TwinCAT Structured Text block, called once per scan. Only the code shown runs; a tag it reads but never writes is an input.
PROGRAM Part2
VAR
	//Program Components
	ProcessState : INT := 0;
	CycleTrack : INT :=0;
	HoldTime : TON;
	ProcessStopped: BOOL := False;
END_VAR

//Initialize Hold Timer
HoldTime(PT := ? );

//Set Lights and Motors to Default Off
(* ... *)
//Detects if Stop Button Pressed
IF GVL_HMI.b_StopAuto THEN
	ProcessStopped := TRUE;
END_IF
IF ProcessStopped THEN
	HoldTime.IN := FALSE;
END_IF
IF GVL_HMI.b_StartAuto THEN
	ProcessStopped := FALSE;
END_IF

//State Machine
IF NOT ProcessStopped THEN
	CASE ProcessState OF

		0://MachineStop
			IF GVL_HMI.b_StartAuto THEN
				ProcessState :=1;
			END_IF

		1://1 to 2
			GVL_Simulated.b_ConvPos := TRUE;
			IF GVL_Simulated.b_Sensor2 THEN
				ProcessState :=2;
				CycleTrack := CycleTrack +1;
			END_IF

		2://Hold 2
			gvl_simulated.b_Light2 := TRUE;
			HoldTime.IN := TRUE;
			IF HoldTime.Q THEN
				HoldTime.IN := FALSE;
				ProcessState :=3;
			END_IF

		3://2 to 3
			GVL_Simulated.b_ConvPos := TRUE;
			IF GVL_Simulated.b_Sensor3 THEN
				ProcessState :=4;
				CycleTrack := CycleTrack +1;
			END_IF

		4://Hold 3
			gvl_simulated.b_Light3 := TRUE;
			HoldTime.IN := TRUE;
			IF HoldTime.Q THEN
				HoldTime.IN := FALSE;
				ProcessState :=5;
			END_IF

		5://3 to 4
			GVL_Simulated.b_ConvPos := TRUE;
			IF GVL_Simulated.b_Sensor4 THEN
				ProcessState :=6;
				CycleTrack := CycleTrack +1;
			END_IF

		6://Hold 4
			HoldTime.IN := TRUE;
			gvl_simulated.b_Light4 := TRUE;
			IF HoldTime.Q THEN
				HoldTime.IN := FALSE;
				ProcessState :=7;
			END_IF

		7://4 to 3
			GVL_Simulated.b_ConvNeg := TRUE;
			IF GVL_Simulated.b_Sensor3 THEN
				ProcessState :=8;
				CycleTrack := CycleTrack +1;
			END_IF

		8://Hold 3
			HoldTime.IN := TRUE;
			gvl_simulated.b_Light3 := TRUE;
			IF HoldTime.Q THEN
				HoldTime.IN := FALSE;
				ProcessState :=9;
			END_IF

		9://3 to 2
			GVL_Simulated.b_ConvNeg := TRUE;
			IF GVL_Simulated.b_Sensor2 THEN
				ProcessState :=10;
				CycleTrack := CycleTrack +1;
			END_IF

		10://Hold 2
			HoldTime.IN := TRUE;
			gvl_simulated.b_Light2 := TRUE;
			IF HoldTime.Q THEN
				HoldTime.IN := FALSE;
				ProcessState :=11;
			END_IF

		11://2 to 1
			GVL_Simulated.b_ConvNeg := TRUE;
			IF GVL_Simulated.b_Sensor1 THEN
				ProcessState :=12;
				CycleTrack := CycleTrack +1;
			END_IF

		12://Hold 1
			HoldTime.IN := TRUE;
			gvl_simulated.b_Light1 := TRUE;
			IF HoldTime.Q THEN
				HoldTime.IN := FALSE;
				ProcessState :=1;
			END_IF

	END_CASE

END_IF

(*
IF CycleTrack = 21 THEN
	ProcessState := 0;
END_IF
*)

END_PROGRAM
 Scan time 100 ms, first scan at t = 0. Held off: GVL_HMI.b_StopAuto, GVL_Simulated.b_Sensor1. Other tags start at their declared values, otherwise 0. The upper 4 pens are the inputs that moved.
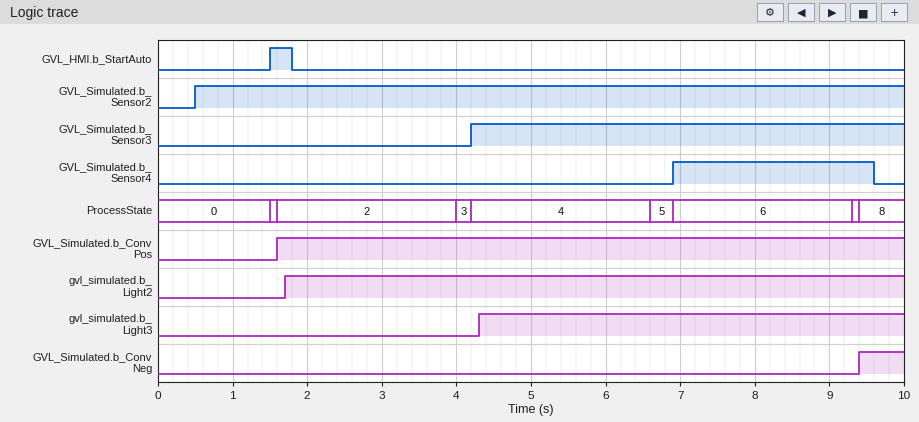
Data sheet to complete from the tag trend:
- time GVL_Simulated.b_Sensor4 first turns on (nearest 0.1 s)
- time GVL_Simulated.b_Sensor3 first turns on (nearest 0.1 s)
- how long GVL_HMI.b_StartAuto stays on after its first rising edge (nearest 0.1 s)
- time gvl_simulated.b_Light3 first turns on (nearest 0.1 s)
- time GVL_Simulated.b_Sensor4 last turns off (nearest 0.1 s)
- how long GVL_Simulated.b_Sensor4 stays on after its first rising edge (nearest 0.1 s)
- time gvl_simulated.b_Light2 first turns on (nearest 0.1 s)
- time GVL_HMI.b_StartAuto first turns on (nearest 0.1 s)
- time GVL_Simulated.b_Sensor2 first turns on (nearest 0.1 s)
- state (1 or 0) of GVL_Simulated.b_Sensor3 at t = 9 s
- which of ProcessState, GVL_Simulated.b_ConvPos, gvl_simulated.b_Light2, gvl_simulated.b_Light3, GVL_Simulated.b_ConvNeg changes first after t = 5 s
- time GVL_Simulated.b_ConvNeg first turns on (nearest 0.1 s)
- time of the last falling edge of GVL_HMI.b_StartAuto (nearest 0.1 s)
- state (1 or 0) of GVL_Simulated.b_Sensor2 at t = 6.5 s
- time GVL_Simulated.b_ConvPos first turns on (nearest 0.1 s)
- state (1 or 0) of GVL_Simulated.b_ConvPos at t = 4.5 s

6.9 s
4.2 s
0.3 s
4.3 s
9.6 s
2.7 s
1.7 s
1.5 s
0.5 s
1
ProcessState
9.4 s
1.8 s
1
1.6 s
1
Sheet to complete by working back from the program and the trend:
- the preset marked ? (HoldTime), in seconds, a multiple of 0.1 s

2.2 s
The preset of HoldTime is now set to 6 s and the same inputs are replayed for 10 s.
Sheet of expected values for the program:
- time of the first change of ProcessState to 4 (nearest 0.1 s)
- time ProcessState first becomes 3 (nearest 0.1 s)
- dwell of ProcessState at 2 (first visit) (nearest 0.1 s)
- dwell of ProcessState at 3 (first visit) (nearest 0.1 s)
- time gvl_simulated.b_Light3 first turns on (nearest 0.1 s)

7.9 s
7.8 s
6.2 s
0.1 s
8.0 s
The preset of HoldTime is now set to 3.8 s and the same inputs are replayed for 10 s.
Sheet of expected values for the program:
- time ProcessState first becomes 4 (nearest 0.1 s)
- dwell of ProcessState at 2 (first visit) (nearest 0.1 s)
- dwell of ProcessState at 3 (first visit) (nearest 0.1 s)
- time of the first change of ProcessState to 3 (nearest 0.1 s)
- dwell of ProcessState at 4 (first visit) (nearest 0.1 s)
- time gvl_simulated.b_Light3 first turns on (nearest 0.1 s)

5.7 s
4.0 s
0.1 s
5.6 s
4.0 s
5.8 s
